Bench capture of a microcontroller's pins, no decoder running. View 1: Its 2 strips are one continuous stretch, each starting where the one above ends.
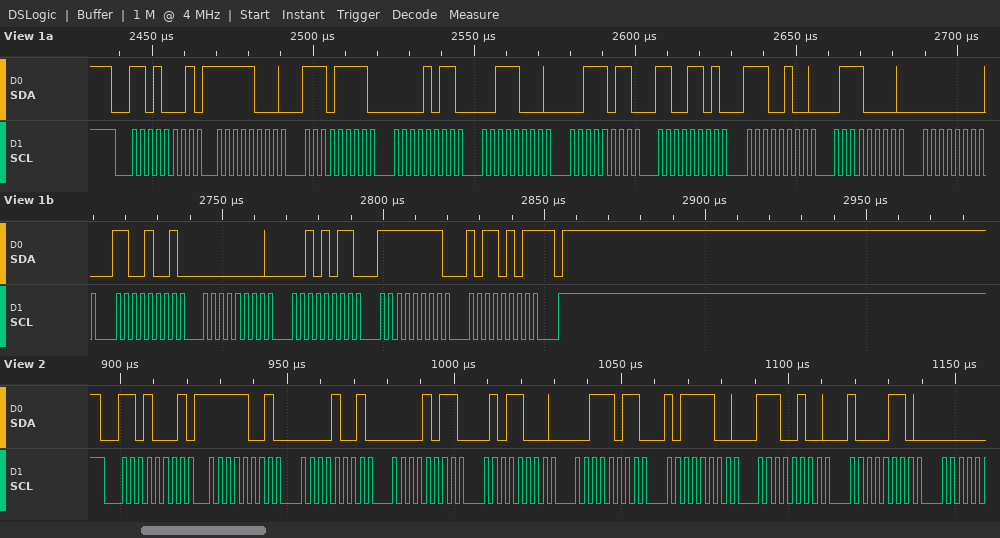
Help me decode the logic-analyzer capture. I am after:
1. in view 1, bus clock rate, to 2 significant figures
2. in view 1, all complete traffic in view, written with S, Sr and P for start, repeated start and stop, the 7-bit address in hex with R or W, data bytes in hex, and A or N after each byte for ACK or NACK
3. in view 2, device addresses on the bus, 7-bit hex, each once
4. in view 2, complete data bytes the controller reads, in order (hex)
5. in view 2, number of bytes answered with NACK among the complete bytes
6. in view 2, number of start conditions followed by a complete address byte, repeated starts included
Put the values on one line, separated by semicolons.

400 kHz; S 68R A F8 A EF A 0B A 38 A 3B A CD A E4 A 70 A 00 A C9 A 00 A 2B A FF A B5 N P; 0x68; F9 09 0B 58 3B BC E4 86; 0; 1
